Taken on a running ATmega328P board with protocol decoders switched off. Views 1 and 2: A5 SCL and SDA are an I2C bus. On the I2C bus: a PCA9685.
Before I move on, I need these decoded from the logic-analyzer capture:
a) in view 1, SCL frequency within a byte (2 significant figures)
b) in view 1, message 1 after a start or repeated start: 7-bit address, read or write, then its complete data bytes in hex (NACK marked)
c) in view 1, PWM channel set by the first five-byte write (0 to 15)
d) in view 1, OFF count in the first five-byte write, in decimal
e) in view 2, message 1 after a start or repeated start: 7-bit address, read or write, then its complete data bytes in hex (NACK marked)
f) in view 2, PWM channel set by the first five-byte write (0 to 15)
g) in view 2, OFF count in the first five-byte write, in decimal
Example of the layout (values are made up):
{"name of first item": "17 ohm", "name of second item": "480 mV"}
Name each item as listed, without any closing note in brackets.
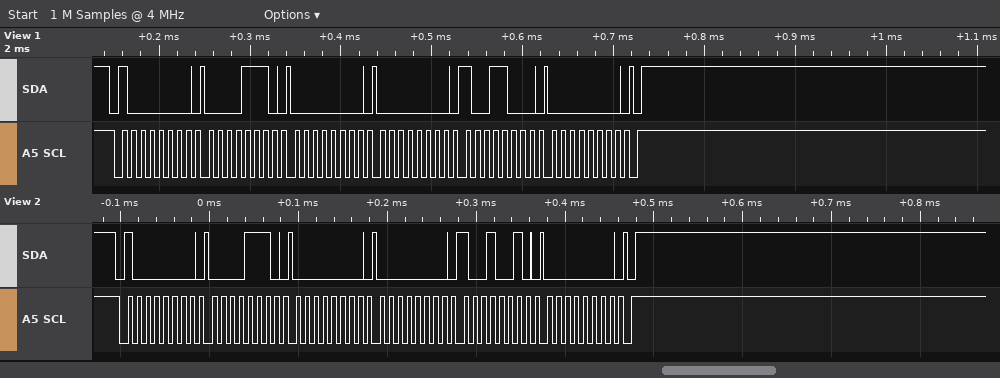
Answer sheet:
{"in view 1, SCL frequency within a byte": "100 kHz", "in view 1, message 1 after a start or repeated start: 7-bit address, read or write, then its complete data bytes in hex": "0x40 write: 0E 00 00 98 00", "in view 1, PWM channel set by the first five-byte write": "2", "in view 1, OFF count in the first five-byte write, in decimal": "152", "in view 2, message 1 after a start or repeated start: 7-bit address, read or write, then its complete data bytes in hex": "0x40 write: 0E 00 00 92 00", "in view 2, PWM channel set by the first five-byte write": "2", "in view 2, OFF count in the first five-byte write, in decimal": "146"}
